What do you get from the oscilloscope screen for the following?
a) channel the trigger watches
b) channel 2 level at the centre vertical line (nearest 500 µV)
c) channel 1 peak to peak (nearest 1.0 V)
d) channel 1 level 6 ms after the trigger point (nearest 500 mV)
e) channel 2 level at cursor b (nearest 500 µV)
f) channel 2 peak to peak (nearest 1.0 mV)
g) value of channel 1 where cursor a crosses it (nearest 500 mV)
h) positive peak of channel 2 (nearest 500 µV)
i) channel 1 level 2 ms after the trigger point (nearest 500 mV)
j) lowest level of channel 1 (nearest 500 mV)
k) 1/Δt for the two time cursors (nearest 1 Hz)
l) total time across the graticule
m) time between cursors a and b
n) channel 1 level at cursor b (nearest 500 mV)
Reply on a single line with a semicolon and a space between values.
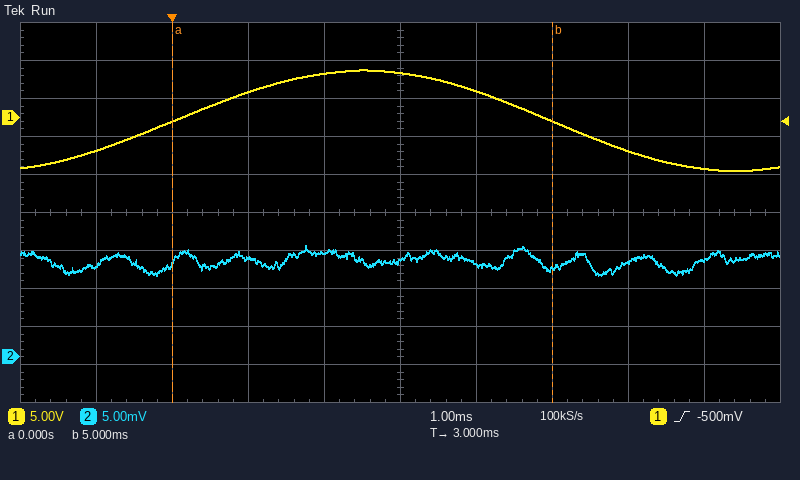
channel 1; 12.5 mV; 13.0 V; -4.5 V; 11.5 mV; 4.0 mV; -500 mV; 14.5 mV; 6.0 V; -7.0 V; 200 Hz; 10 ms; 5.0 ms; -500 mV
